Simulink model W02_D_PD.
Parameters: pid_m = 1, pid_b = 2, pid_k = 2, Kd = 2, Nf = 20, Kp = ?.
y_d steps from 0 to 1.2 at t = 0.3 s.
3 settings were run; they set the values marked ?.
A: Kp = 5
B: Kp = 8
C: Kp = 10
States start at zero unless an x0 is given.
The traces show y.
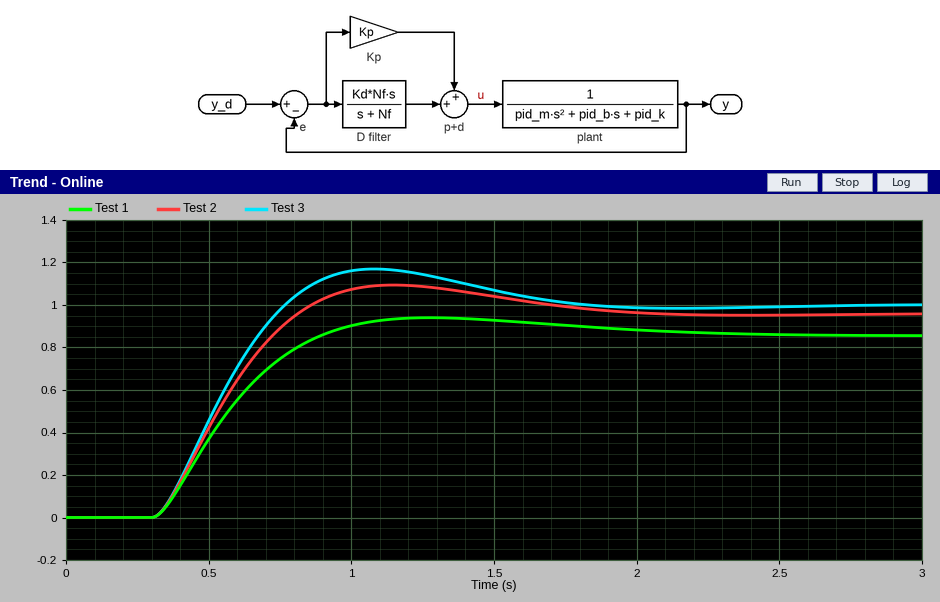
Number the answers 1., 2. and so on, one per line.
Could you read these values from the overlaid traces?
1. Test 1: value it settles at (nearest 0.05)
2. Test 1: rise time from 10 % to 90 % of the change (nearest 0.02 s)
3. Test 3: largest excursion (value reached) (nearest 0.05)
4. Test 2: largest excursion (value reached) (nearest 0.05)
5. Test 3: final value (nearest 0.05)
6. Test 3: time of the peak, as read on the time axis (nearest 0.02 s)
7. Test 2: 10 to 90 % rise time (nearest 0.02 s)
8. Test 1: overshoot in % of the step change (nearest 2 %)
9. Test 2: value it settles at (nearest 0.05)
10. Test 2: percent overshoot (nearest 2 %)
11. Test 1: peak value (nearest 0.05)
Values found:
1. 0.85
2. 0.40 s
3. 1.15
4. 1.10
5. 1.00
6. 1.08 s
7. 0.36 s
8. 10 %
9. 0.95
10. 14 %
11. 0.95
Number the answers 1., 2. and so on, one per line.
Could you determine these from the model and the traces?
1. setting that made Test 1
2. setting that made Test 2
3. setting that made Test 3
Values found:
1. A
2. B
3. C
